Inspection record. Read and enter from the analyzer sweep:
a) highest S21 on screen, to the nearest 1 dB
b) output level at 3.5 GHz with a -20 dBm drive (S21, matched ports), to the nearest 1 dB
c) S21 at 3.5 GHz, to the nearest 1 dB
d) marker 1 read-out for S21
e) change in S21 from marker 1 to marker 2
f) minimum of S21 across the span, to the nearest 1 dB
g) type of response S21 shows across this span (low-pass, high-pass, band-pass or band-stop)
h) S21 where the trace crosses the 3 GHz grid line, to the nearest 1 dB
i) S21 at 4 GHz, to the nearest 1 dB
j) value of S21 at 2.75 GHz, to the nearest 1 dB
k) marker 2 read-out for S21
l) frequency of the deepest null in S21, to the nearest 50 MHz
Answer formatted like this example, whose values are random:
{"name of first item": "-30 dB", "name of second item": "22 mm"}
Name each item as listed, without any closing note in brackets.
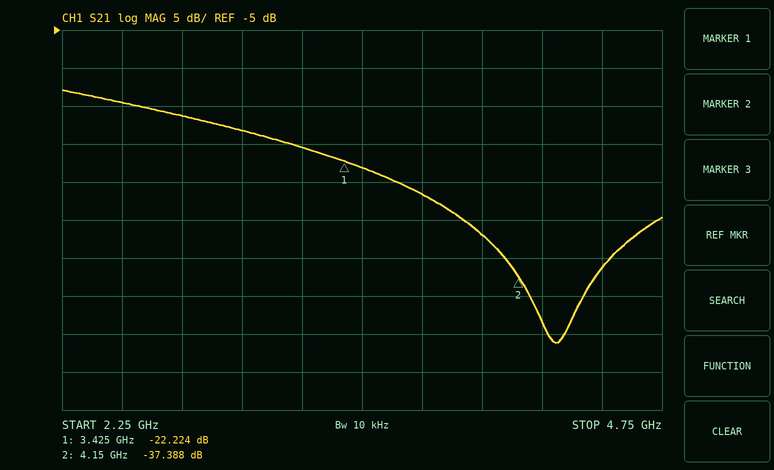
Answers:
{"highest S21 on screen, to the nearest 1 dB": "-13 dB", "output level at 3.5 GHz with a -20 dBm drive (S21, matched ports), to the nearest 1 dB": "-43 dBm", "S21 at 3.5 GHz, to the nearest 1 dB": "-23 dB", "marker 1 read-out for S21": "-22.224 dB", "change in S21 from marker 1 to marker 2": "-15.164 dB", "minimum of S21 across the span, to the nearest 1 dB": "-46 dB", "type of response S21 shows across this span": "low-pass", "S21 where the trace crosses the 3 GHz grid line, to the nearest 1 dB": "-18 dB", "S21 at 4 GHz, to the nearest 1 dB": "-32 dB", "value of S21 at 2.75 GHz, to the nearest 1 dB": "-16 dB", "marker 2 read-out for S21": "-37.388 dB", "frequency of the deepest null in S21, to the nearest 50 MHz": "4.30 GHz"}
